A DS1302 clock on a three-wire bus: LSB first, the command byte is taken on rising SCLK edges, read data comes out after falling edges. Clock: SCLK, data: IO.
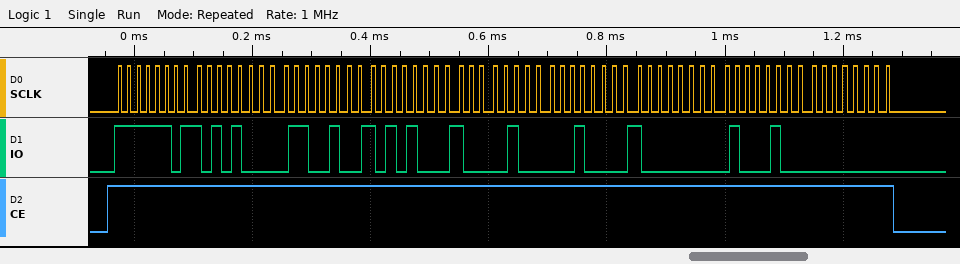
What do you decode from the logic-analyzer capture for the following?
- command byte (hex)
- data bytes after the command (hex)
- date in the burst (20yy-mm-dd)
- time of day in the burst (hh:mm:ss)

0xBF
15 26 15 21 08 01 22 00
2022-08-21
15:26:15
